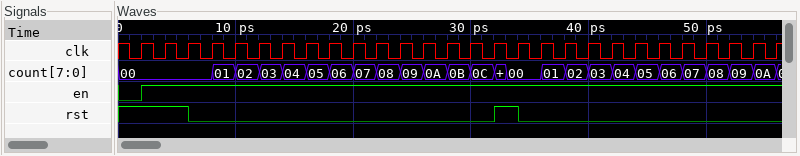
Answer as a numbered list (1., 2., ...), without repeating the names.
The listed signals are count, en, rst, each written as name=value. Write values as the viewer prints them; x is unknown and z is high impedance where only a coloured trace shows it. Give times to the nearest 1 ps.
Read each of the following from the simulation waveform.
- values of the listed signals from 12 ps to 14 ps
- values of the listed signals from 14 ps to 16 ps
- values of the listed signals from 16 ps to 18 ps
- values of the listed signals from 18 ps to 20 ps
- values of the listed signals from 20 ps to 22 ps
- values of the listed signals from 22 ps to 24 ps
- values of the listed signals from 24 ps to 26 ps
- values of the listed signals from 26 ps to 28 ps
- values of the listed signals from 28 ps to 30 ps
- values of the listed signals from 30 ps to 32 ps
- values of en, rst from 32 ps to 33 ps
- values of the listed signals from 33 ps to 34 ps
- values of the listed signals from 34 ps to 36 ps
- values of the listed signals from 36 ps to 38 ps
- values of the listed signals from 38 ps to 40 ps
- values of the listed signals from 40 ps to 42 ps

1. count=03, en=1, rst=0
2. count=04, en=1, rst=0
3. count=05, en=1, rst=0
4. count=06, en=1, rst=0
5. count=07, en=1, rst=0
6. count=08, en=1, rst=0
7. count=09, en=1, rst=0
8. count=0A, en=1, rst=0
9. count=0B, en=1, rst=0
10. count=0C, en=1, rst=0
11. en=1, rst=1
12. count=00, en=1, rst=1
13. count=00, en=1, rst=0
14. count=01, en=1, rst=0
15. count=02, en=1, rst=0
16. count=03, en=1, rst=0
